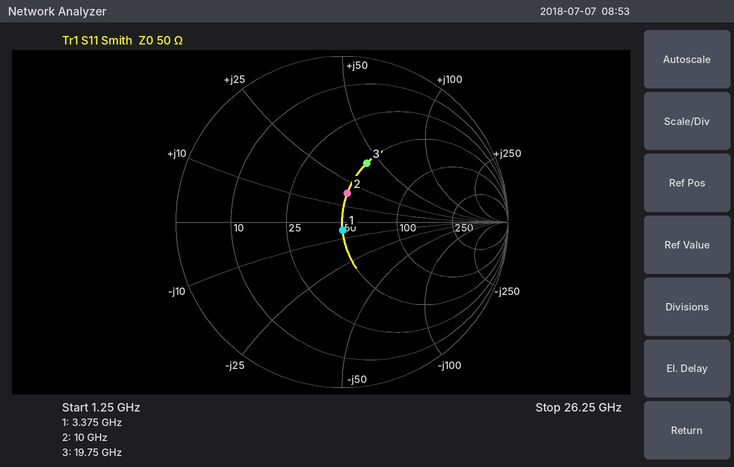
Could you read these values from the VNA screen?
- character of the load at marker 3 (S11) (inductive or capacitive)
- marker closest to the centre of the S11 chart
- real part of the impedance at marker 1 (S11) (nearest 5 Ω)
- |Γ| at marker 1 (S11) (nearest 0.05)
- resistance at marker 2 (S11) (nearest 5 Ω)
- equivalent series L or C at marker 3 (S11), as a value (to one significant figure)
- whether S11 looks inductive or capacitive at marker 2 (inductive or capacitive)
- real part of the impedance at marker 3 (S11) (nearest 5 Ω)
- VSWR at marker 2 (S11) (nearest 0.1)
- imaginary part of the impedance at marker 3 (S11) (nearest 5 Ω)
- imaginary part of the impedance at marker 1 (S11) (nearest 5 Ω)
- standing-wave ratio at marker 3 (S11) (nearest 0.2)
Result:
inductive
marker 1
50 Ω
0.05
50 Ω
300 pH
inductive
50 Ω
1.4
+40 Ω
-5 Ω
2.2
